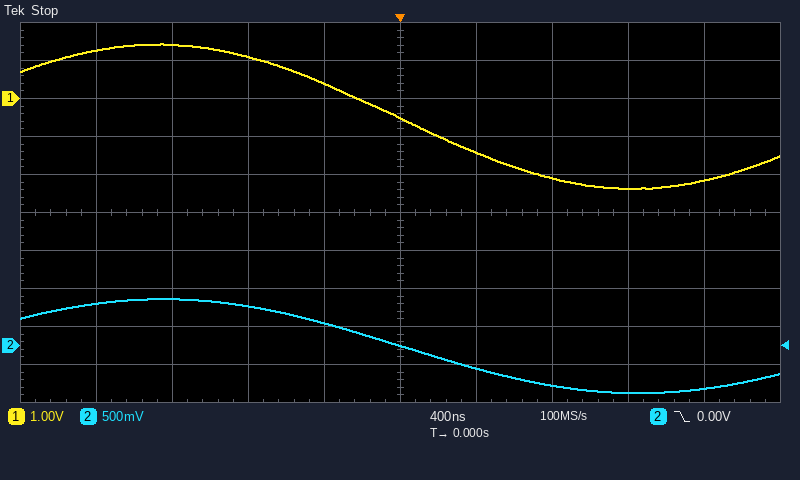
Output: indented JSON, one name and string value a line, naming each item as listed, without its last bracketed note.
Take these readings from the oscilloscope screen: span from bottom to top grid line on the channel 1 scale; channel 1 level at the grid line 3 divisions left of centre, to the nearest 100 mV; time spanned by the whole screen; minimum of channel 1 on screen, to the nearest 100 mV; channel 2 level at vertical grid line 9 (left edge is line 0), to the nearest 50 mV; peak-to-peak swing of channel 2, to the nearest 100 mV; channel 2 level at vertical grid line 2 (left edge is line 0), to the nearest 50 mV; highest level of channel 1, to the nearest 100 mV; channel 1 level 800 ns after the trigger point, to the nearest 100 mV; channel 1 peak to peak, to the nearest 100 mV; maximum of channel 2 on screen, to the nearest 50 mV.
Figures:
{
  "span from bottom to top grid line on the channel 1 scale": "10 V",
  "channel 1 level at the grid line 3 divisions left of centre, to the nearest 100 mV": "1.4 V",
  "time spanned by the whole screen": "4 µs",
  "minimum of channel 1 on screen, to the nearest 100 mV": "-2.4 V",
  "channel 2 level at vertical grid line 9 (left edge is line 0), to the nearest 50 mV": "-550 mV",
  "peak-to-peak swing of channel 2, to the nearest 100 mV": "1.20 V",
  "channel 2 level at vertical grid line 2 (left edge is line 0), to the nearest 50 mV": "600 mV",
  "highest level of channel 1, to the nearest 100 mV": "1.4 V",
  "channel 1 level 800 ns after the trigger point, to the nearest 100 mV": "-2.1 V",
  "channel 1 peak to peak, to the nearest 100 mV": "3.8 V",
  "maximum of channel 2 on screen, to the nearest 50 mV": "600 mV"
}
